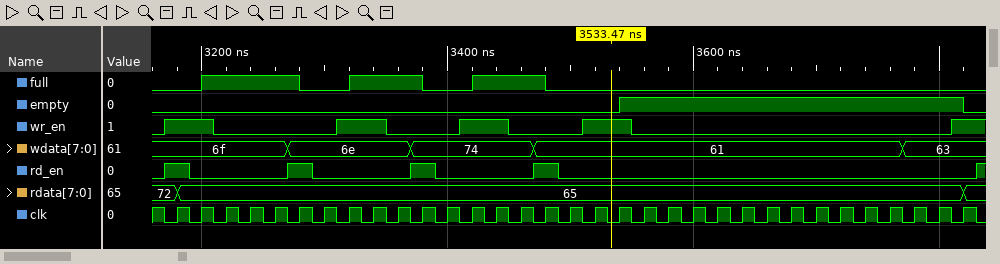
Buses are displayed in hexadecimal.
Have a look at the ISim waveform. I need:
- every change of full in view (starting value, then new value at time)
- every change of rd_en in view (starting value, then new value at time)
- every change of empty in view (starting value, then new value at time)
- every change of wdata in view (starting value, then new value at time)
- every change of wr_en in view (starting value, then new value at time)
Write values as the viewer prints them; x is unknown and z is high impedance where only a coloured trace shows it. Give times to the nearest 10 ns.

0, 1 at 3200 ns, 0 at 3280 ns, 1 at 3320 ns, 0 at 3380 ns, 1 at 3420 ns, 0 at 3480 ns
0, 1 at 3170 ns, 0 at 3190 ns, 1 at 3270 ns, 0 at 3290 ns, 1 at 3370 ns, 0 at 3390 ns, 1 at 3470 ns, 0 at 3490 ns, 1 at 3830 ns
0, 1 at 3540 ns, 0 at 3820 ns
6f, 6e at 3270 ns, 74 at 3370 ns, 61 at 3470 ns, 63 at 3770 ns
0, 1 at 3170 ns, 0 at 3210 ns, 1 at 3310 ns, 0 at 3350 ns, 1 at 3410 ns, 0 at 3450 ns, 1 at 3510 ns, 0 at 3550 ns, 1 at 3810 ns
